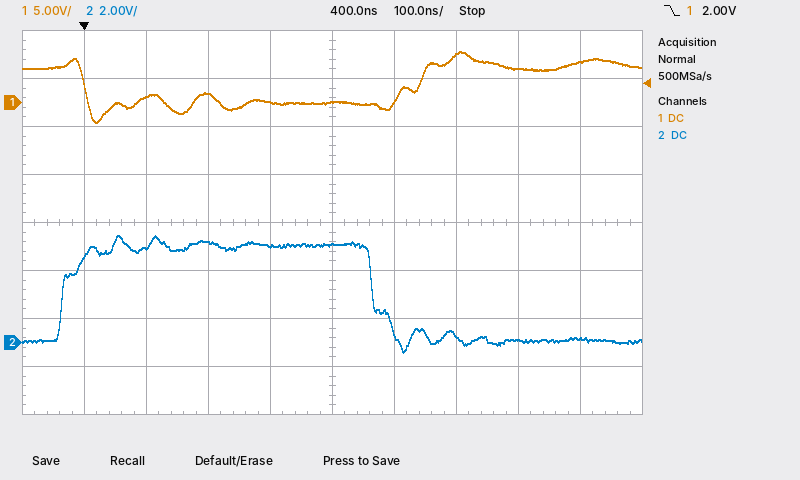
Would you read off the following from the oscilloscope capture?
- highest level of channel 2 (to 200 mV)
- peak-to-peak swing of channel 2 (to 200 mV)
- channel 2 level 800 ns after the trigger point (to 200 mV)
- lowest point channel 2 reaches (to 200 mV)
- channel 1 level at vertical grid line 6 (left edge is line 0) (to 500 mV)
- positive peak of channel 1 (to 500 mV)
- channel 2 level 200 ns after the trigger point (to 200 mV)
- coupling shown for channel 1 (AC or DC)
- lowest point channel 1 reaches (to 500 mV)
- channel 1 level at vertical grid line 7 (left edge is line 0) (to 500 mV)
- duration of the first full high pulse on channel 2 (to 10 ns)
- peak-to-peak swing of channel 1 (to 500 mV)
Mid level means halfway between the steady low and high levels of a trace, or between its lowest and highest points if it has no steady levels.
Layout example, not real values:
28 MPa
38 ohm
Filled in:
4.4 V
4.8 V
200 mV
-400 mV
0.0 V
5.5 V
4.2 V
DC
-2.0 V
5.0 V
500 ns
7.5 V
